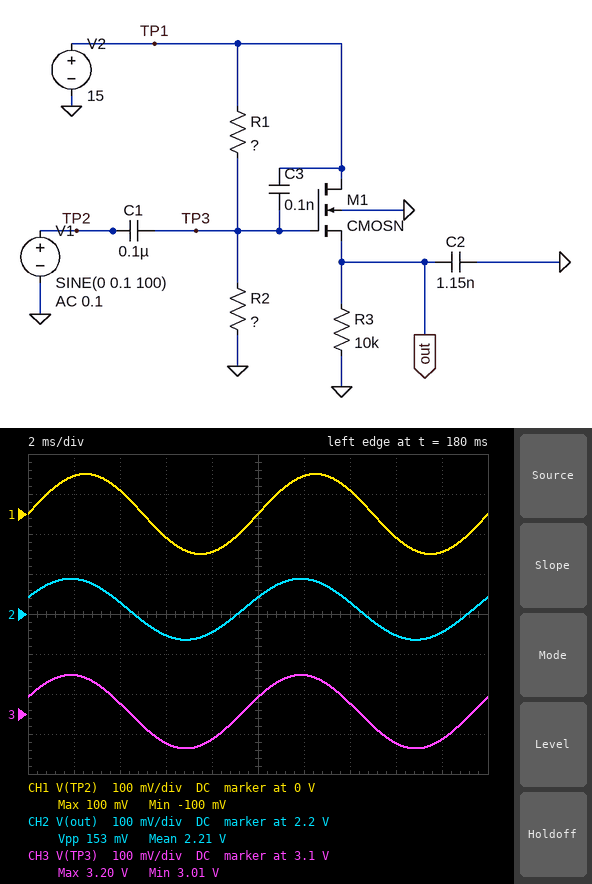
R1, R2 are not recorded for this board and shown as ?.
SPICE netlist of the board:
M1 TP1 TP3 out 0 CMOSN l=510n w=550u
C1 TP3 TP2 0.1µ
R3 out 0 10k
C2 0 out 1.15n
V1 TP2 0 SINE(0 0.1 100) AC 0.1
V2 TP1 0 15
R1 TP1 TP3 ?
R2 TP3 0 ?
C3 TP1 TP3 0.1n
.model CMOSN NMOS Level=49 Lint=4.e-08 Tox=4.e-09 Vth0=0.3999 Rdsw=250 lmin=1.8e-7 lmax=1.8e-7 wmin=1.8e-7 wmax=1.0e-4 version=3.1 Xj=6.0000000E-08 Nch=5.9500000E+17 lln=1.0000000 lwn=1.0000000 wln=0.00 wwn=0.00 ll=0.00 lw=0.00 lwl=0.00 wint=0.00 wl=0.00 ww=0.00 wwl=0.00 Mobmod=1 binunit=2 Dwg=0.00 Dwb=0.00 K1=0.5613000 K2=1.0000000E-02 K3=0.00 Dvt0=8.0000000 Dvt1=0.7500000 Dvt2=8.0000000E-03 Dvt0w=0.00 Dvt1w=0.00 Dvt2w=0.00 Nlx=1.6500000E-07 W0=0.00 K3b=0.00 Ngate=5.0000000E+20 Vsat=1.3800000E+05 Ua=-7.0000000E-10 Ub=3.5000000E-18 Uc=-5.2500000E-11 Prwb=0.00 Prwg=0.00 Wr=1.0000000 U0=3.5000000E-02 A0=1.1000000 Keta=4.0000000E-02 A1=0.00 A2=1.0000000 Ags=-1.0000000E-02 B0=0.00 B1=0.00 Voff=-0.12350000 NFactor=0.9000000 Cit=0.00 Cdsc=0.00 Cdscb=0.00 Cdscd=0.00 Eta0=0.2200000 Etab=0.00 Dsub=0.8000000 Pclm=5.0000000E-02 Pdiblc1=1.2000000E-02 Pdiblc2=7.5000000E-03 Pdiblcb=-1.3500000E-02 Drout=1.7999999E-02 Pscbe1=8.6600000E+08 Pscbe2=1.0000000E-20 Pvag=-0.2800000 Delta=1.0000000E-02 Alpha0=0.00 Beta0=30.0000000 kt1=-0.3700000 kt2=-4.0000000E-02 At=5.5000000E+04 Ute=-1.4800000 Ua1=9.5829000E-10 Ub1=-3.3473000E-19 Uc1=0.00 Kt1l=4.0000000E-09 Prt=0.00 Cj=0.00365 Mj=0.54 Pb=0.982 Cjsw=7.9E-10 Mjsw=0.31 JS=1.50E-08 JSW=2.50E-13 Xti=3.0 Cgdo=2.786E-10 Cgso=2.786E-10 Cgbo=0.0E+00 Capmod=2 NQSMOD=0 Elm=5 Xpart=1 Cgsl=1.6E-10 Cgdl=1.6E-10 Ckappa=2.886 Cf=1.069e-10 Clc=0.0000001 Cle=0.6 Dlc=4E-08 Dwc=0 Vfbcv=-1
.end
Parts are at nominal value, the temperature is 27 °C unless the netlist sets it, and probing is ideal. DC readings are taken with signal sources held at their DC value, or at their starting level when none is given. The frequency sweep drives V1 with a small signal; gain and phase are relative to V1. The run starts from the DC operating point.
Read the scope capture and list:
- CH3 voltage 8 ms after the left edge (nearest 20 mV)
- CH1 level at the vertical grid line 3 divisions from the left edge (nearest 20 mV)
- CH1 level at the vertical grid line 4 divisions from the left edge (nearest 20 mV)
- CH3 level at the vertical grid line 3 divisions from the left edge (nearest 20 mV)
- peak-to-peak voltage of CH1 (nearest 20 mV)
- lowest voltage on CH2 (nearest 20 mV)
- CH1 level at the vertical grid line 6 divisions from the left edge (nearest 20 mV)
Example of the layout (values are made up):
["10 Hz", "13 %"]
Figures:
["3.04 V", "-60 mV", "-100 mV", "3.02 V", "200 mV", "2.14 V", "100 mV"]
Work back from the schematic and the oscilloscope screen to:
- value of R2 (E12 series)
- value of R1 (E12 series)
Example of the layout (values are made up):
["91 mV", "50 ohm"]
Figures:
["47 kΩ", "180 kΩ"]
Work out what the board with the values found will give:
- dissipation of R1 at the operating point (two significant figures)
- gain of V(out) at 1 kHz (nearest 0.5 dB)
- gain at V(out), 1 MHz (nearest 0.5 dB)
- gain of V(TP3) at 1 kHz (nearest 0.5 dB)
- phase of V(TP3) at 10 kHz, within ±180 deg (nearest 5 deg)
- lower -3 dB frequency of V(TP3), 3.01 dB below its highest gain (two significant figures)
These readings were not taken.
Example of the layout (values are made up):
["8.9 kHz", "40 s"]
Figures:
["790 µW", "-1.5 dB", "-5.5 dB", "0 dB", "0 deg", "43 Hz"]
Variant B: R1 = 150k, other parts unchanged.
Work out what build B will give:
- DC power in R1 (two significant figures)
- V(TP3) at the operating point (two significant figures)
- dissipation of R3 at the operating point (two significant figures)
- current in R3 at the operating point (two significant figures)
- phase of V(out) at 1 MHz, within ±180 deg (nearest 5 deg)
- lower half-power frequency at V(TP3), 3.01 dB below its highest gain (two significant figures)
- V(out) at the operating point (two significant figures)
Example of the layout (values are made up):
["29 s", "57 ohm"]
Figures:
["870 µW", "3.6 V", "680 µW", "260 µA", "-45 deg", "44 Hz", "2.6 V"]
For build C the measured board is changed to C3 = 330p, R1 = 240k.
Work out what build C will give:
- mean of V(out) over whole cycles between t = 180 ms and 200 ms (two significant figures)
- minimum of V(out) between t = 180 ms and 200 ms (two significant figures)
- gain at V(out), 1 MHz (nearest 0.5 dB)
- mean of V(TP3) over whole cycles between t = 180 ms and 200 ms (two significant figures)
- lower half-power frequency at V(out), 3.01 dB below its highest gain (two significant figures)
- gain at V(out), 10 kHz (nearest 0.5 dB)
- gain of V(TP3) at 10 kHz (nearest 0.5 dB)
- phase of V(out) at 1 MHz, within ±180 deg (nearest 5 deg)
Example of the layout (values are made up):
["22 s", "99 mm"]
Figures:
["1.7 V", "1.6 V", "-7.0 dB", "2.5 V", "40 Hz", "-2.0 dB", "0 dB", "-55 deg"]
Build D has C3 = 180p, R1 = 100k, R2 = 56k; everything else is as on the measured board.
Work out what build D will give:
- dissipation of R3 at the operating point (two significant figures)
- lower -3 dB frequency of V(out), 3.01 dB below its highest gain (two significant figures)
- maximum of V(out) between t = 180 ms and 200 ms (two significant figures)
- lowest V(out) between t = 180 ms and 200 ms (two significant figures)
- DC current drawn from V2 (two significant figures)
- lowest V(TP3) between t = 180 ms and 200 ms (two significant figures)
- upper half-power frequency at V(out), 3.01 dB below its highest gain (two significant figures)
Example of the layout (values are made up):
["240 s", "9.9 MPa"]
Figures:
["1.7 mW", "44 Hz", "4.2 V", "4.1 V", "510 µA", "5.3 V", "1.3 MHz"]
